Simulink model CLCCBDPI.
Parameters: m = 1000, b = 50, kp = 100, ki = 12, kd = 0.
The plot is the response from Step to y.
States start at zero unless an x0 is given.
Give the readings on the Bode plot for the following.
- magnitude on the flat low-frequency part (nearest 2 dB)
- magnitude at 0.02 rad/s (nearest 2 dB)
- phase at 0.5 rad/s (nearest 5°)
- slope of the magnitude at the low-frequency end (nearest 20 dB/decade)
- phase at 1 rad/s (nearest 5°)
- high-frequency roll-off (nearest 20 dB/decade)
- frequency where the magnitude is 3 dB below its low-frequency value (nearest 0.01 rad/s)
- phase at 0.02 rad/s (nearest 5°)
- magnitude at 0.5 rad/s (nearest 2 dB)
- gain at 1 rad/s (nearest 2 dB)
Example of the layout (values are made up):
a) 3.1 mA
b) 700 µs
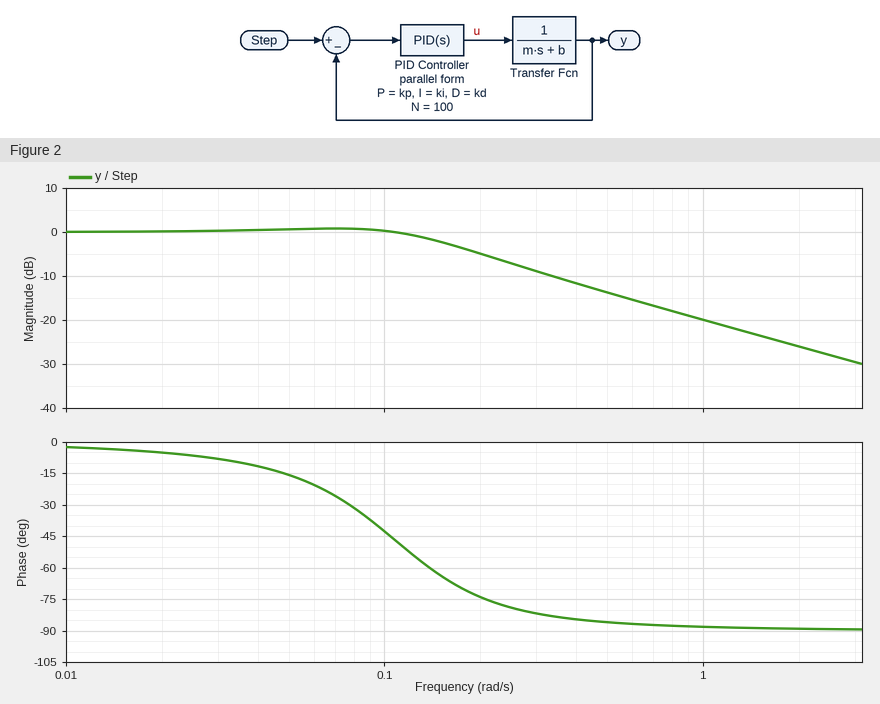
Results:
a) 0 dB
b) 0 dB
c) -85°
d) 0 dB/decade
e) -90°
f) -20 dB/decade
g) 0.16 rad/s
h) -5°
i) -14 dB
j) -20 dB
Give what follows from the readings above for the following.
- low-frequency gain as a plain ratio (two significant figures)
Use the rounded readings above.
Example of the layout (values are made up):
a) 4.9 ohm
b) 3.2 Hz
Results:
a) 1.0
